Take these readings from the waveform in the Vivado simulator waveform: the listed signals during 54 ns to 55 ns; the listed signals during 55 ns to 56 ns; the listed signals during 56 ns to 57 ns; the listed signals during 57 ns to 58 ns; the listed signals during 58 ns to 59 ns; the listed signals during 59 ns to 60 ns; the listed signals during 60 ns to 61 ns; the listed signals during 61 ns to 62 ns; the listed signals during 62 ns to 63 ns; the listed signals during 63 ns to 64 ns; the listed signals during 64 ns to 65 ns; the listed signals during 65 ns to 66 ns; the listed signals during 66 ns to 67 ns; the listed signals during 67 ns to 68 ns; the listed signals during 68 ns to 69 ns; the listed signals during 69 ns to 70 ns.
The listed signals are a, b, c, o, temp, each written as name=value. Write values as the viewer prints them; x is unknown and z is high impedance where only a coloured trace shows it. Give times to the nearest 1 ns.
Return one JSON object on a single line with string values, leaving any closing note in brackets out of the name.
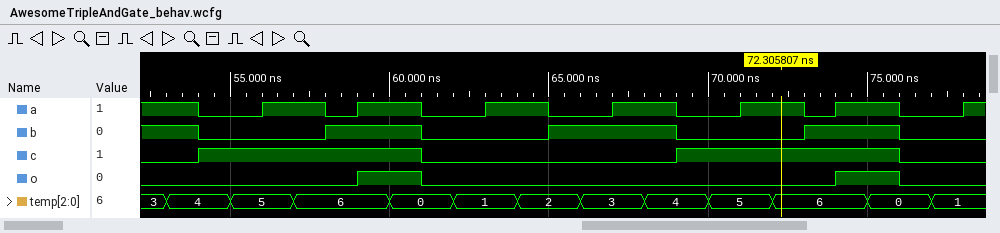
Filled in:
{"the listed signals during 54 ns to 55 ns": "a=0, b=0, c=1, o=0, temp=4", "the listed signals during 55 ns to 56 ns": "a=0, b=0, c=1, o=0, temp=5", "the listed signals during 56 ns to 57 ns": "a=1, b=0, c=1, o=0, temp=5", "the listed signals during 57 ns to 58 ns": "a=1, b=0, c=1, o=0, temp=6", "the listed signals during 58 ns to 59 ns": "a=0, b=1, c=1, o=0, temp=6", "the listed signals during 59 ns to 60 ns": "a=1, b=1, c=1, o=1, temp=6", "the listed signals during 60 ns to 61 ns": "a=1, b=1, c=1, o=1, temp=0", "the listed signals during 61 ns to 62 ns": "a=0, b=0, c=0, o=0, temp=0", "the listed signals during 62 ns to 63 ns": "a=0, b=0, c=0, o=0, temp=1", "the listed signals during 63 ns to 64 ns": "a=1, b=0, c=0, o=0, temp=1", "the listed signals during 64 ns to 65 ns": "a=1, b=0, c=0, o=0, temp=2", "the listed signals during 65 ns to 66 ns": "a=0, b=1, c=0, o=0, temp=2", "the listed signals during 66 ns to 67 ns": "a=0, b=1, c=0, o=0, temp=3", "the listed signals during 67 ns to 68 ns": "a=1, b=1, c=0, o=0, temp=3", "the listed signals during 68 ns to 69 ns": "a=1, b=1, c=0, o=0, temp=4", "the listed signals during 69 ns to 70 ns": "a=0, b=0, c=1, o=0, temp=4"}
